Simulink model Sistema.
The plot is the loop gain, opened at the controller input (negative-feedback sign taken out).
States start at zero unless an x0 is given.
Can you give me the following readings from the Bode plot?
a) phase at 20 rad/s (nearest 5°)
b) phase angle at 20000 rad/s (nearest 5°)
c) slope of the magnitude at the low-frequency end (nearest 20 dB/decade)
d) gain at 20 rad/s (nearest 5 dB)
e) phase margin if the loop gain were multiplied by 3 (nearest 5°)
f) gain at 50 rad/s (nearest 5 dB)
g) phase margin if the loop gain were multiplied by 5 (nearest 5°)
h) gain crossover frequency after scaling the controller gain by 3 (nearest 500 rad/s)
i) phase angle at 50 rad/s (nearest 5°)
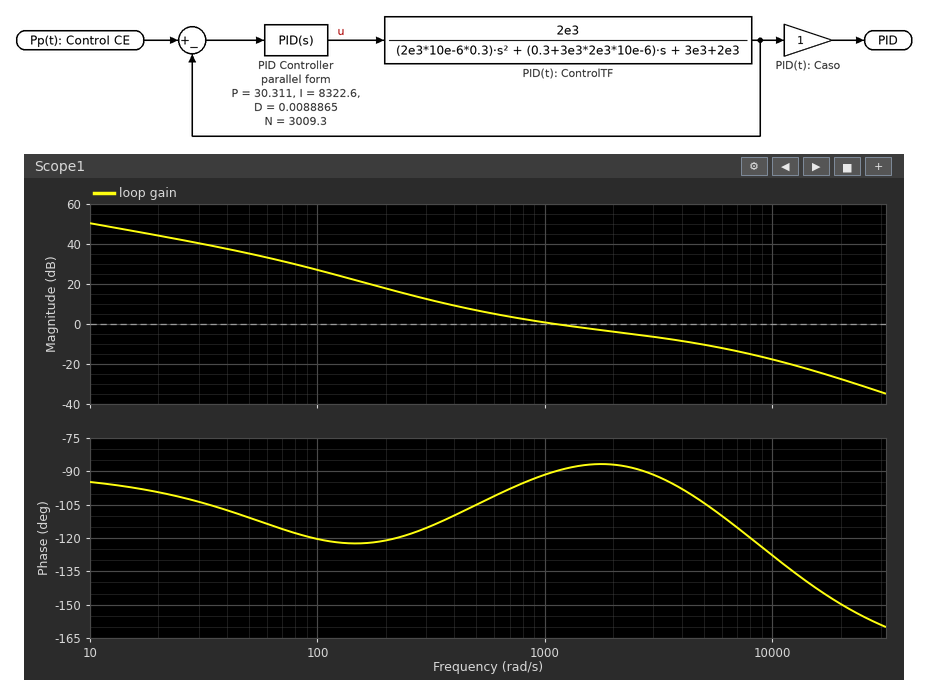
-100°
-150°
-20 dB/decade
45 dB
80°
35 dB
65°
4500 rad/s
-110°
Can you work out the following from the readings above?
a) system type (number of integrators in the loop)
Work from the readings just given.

1
